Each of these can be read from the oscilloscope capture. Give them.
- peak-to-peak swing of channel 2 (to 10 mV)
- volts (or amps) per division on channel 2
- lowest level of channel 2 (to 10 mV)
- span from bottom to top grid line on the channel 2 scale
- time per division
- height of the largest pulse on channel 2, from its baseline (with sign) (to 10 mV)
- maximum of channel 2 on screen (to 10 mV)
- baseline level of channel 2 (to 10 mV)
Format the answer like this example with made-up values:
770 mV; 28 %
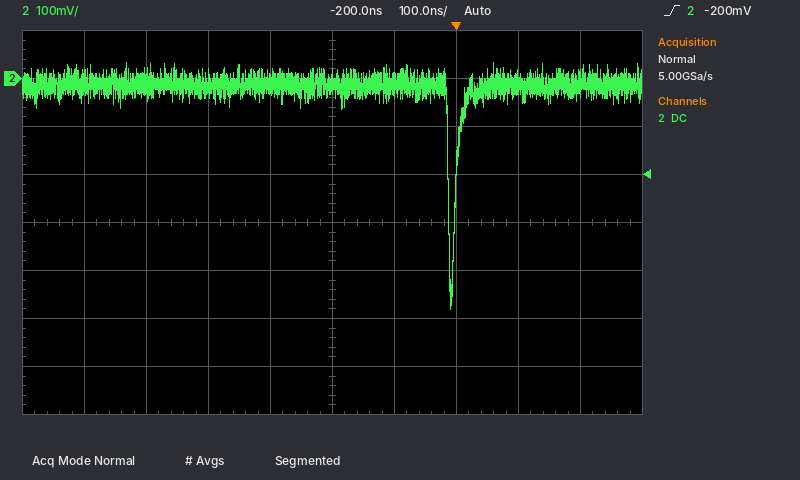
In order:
510 mV; 100 mV; -480 mV; 800 mV; 100 ns; -470 mV; 30 mV; -10 mV
